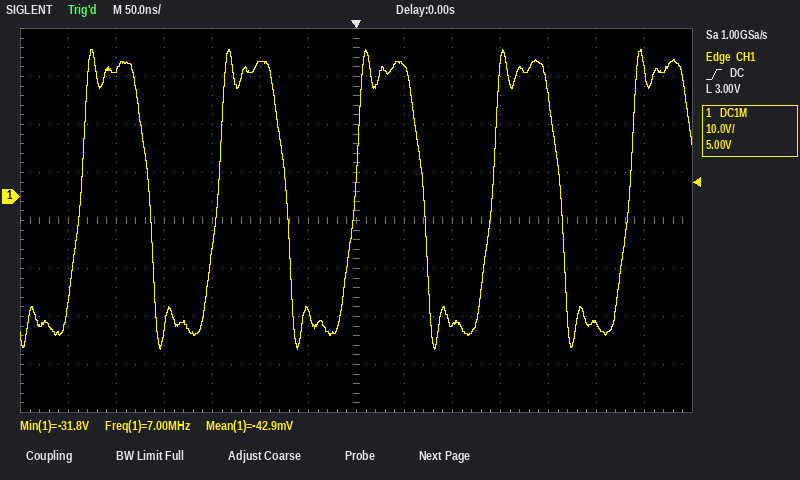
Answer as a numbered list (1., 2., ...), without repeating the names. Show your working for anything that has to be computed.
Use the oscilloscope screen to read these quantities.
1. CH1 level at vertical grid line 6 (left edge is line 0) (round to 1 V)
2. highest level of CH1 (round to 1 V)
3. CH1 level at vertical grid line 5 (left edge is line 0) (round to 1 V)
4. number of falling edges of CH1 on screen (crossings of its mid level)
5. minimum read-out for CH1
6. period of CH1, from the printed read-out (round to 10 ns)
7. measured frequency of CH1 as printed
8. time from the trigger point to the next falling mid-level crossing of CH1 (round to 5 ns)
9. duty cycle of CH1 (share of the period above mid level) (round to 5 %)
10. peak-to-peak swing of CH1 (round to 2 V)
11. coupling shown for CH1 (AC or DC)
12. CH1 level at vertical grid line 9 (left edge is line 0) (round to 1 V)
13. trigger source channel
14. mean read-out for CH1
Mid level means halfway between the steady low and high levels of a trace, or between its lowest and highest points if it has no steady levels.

1. -24 V
2. 31 V
3. 28 V
4. 4
5. -31.8 V
6. 1 / 7.00 MHz ≈ 143 ns, so 140 ns to the nearest 10 ns
7. 7.00 MHz
8. 70 ns
9. 50 %
10. 62 V
11. DC
12. -27 V
13. CH1
14. -42.9 mV
